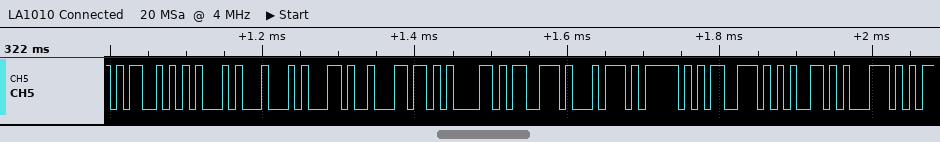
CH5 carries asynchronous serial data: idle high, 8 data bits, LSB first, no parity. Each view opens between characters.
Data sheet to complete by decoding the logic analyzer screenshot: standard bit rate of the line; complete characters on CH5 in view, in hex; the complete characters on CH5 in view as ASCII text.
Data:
115200 baud
4D, 45, 44, 2C, 6C, 61, 73, 74, 5F, 73, 65, 71
"MED,last_seq"
